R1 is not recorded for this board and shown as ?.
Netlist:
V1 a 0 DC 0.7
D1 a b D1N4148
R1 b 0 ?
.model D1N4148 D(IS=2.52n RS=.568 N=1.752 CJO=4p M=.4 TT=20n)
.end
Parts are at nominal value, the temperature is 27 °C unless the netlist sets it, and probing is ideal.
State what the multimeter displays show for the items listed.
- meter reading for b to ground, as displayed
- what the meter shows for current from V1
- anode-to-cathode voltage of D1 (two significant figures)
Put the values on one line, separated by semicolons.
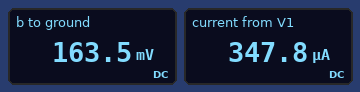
163.5 mV; 347.8 µA; 540 mV
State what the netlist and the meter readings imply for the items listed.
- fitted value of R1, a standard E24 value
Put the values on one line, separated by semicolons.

470 Ω
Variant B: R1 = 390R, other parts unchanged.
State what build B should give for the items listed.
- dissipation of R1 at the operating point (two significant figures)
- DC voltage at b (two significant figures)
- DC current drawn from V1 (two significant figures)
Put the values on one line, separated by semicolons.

63 µW; 160 mV; 400 µA
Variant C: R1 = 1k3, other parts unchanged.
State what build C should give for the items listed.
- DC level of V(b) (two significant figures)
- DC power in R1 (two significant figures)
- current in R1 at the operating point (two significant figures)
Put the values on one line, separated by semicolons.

200 mV; 31 µW; 150 µA
